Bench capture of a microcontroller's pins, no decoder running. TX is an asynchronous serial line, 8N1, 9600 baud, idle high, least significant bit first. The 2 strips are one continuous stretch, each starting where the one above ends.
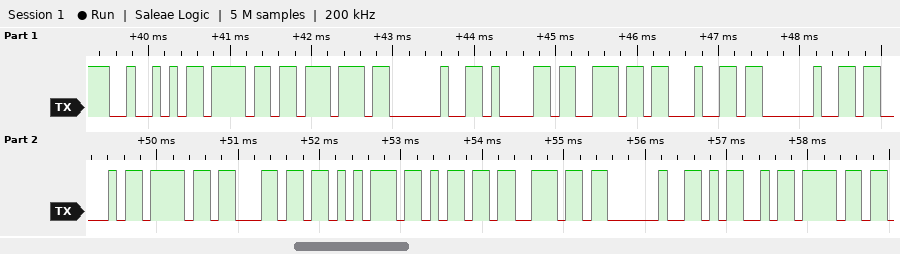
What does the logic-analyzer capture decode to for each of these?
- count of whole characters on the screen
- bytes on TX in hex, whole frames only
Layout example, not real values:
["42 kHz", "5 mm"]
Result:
["17", "0x52 0x6F 0x77 0x20 0x61 0x6E 0x64 0x20 0x43 0x6F 0x6C 0x75 0x6D 0x6E 0x20 0x4D 0x6F"]
